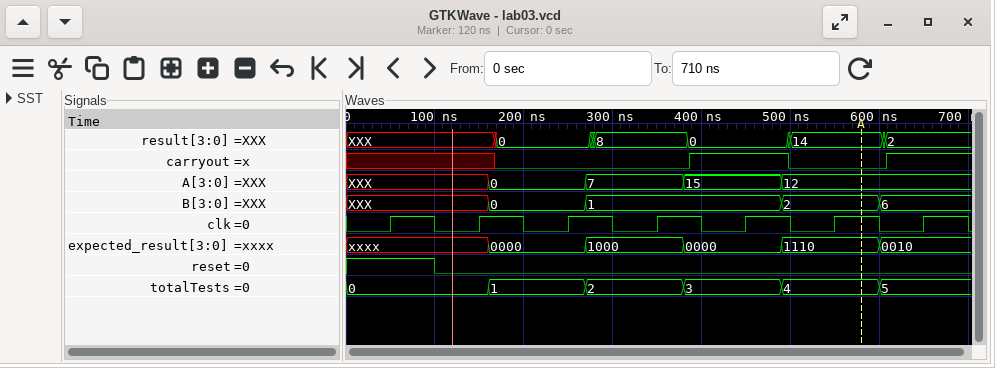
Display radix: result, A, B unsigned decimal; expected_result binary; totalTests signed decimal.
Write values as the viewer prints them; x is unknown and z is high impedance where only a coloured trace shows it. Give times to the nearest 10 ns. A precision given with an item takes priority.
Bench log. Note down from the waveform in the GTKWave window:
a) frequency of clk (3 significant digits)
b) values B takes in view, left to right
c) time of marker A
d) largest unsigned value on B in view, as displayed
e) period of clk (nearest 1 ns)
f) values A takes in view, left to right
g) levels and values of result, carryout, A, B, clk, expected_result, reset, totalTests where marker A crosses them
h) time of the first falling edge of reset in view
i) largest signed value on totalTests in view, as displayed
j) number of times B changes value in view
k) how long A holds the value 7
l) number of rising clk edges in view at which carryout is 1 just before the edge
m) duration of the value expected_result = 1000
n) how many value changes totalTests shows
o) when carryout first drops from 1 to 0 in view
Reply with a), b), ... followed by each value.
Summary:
a) 10.0 MHz
b) XXX, 0, 1, 2, 6
c) 580 ns
d) 6
e) 100 ns
f) XXX, 0, 7, 15, 12
g) result=14, carryout=0, A=12, B=2, clk=1, expected_result=1110, reset=0, totalTests=4
h) 100 ns
i) 5
j) 4
k) 110 ns
l) 2
m) 110 ns
n) 5
o) 500 ns
